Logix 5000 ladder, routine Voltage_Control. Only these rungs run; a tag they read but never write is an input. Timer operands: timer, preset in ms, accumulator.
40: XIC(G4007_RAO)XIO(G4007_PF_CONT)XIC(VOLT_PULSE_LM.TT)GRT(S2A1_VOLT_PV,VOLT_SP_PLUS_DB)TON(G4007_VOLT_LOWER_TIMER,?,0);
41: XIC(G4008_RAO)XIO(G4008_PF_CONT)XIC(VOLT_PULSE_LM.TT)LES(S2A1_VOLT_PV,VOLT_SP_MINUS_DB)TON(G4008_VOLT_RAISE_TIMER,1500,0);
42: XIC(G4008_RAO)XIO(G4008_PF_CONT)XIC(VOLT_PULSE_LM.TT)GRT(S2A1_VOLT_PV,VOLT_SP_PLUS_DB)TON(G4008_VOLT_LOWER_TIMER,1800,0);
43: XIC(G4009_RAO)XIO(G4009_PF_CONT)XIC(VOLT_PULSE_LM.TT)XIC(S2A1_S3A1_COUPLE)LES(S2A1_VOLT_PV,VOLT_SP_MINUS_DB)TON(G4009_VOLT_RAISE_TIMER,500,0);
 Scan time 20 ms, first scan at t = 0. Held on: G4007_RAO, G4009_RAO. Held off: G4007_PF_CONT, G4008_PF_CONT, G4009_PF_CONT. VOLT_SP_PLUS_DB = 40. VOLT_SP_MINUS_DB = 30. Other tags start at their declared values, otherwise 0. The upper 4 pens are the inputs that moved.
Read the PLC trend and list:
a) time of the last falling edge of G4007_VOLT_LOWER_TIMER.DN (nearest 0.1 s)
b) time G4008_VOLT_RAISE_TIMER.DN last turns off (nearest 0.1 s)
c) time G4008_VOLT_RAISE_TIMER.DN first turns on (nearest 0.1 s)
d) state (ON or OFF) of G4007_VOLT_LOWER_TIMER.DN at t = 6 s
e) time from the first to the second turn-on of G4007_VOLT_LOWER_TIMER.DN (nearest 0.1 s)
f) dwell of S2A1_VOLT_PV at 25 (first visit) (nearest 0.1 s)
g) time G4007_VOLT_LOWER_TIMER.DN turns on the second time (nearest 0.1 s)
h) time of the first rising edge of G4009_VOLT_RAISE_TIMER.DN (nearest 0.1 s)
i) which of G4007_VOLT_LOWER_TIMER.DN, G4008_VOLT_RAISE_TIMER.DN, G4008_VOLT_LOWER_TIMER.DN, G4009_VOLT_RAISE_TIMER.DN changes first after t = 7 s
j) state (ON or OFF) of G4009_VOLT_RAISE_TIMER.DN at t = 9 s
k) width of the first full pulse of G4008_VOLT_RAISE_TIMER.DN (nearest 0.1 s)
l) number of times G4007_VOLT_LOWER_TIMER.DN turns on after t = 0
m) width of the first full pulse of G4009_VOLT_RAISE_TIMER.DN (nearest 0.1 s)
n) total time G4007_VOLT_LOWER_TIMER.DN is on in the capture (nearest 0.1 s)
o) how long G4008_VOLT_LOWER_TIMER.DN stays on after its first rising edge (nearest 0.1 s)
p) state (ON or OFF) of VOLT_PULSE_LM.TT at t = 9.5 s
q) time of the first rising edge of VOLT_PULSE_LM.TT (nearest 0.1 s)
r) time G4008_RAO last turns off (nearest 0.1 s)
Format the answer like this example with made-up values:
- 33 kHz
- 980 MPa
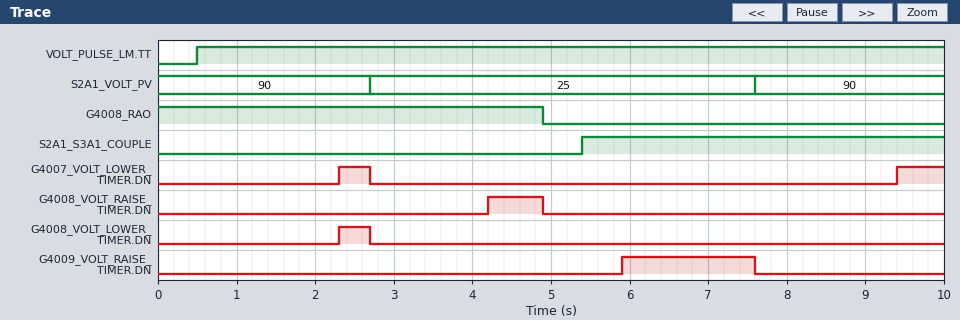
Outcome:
- 2.7 s
- 4.9 s
- 4.2 s
- OFF
- 7.1 s
- 4.9 s
- 9.4 s
- 5.9 s
- G4009_VOLT_RAISE_TIMER.DN
- OFF
- 0.7 s
- 2
- 1.7 s
- 1.0 s
- 0.4 s
- ON
- 0.5 s
- 4.9 s
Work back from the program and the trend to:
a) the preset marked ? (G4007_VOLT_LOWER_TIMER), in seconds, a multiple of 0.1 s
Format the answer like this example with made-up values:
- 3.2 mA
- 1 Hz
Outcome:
- 1.8 s
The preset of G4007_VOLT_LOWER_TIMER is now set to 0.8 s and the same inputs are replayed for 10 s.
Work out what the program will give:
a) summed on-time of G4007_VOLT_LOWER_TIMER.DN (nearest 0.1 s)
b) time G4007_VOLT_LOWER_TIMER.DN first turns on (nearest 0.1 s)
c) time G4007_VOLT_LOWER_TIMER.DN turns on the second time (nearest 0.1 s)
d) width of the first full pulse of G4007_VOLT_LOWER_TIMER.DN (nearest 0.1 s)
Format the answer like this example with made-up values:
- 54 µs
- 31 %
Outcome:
- 3.0 s
- 1.3 s
- 8.4 s
- 1.4 s
